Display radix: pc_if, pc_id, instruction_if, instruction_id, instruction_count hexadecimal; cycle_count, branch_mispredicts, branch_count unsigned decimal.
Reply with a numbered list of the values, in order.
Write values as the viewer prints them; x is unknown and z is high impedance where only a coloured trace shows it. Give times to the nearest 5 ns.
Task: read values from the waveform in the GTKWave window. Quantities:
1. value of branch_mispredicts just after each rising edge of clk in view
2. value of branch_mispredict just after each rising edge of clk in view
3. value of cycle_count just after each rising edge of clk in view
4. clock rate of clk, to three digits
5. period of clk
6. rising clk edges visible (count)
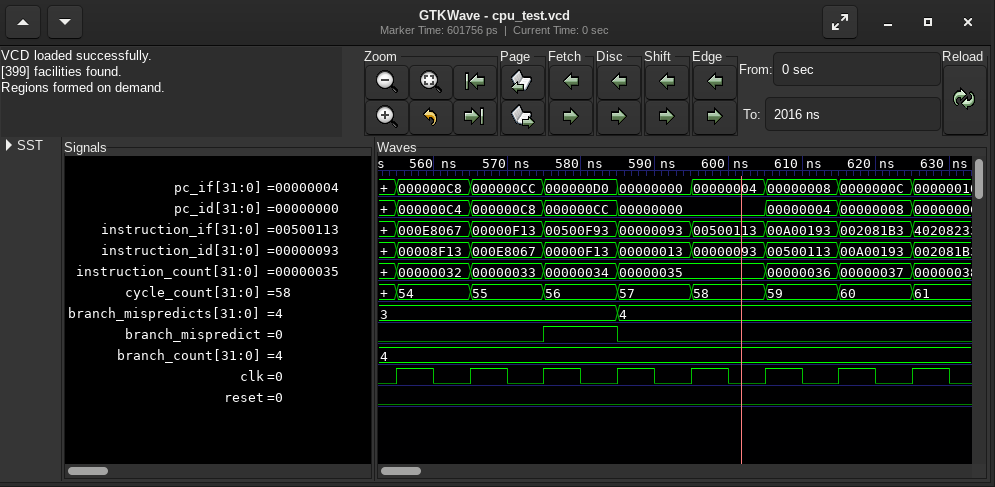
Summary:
1. 3, 3, 3, 4, 4, 4, 4, 4
2. 0 0 1 0 0 0 0 0
3. 54, 55, 56, 57, 58, 59, 60, 61
4. 100 MHz
5. 10 ns
6. 8
